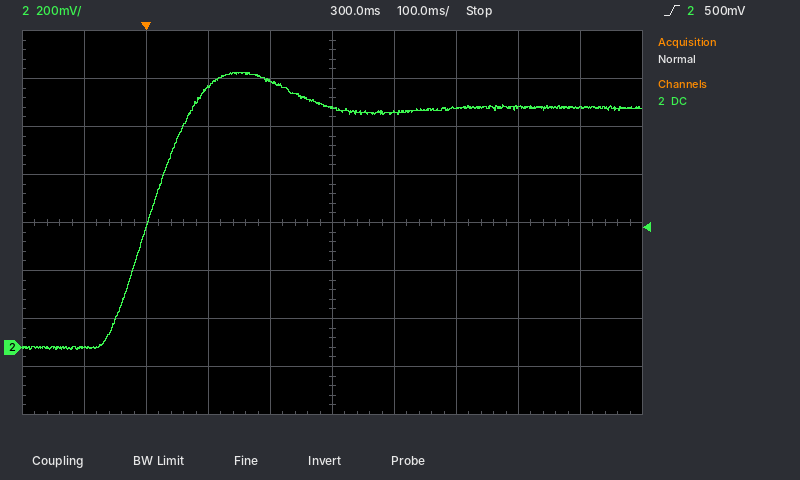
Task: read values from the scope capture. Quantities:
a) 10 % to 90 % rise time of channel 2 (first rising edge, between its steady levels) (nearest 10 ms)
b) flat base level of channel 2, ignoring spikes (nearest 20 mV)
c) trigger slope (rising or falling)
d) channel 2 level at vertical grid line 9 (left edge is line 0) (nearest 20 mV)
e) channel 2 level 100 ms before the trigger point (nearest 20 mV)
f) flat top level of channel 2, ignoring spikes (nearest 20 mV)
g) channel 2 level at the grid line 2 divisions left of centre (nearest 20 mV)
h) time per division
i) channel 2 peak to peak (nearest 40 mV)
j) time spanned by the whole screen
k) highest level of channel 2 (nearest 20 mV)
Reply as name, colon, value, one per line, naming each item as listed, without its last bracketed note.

10 % to 90 % rise time of channel 2 (first rising edge, between its steady levels): 110 ms
flat base level of channel 2, ignoring spikes: 0 mV
trigger slope: rising
channel 2 level at vertical grid line 9 (left edge is line 0): 1.00 V
channel 2 level 100 ms before the trigger point: 0 mV
flat top level of channel 2, ignoring spikes: 1.00 V
channel 2 level at the grid line 2 divisions left of centre: 1.08 V
time per division: 100 ms
channel 2 peak to peak: 1.16 V
time spanned by the whole screen: 1 s
highest level of channel 2: 1.14 V
